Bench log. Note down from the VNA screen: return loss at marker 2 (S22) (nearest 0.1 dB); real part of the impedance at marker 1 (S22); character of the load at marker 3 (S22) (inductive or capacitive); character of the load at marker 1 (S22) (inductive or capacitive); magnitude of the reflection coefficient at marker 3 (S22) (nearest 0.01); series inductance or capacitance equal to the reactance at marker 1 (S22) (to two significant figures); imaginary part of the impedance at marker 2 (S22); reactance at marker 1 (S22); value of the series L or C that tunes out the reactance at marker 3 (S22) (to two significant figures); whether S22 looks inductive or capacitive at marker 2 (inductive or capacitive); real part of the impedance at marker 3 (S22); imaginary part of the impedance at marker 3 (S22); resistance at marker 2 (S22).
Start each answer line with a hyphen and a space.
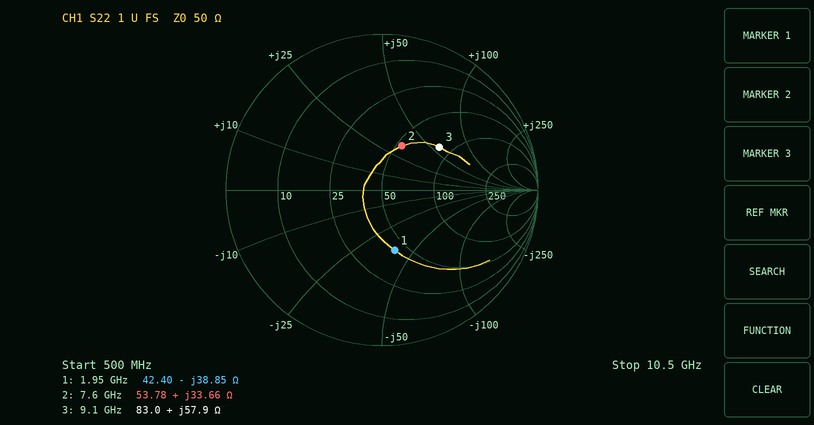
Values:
- 10.2 dB
- 42.40 Ω
- inductive
- capacitive
- 0.46
- 2.1 pF
- +33.66 Ω
- -38.85 Ω
- 300 fF
- inductive
- 83.0 Ω
- +57.9 Ω
- 53.78 Ω
